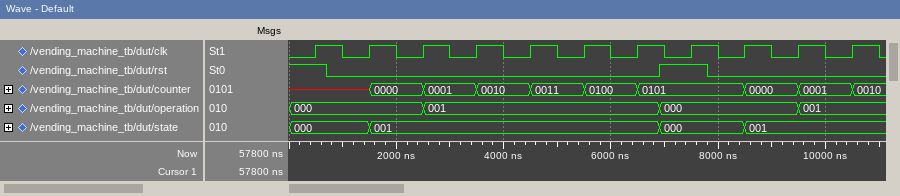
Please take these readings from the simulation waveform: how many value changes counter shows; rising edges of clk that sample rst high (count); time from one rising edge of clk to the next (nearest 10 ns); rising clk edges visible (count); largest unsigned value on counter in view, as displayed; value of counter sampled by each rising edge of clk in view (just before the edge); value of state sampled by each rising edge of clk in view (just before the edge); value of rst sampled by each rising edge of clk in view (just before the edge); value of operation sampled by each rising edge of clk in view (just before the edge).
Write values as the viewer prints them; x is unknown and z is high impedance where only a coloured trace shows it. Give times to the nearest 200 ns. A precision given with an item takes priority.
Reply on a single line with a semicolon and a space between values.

9; 2; 1000 ns; 11; 0101; x, x, 0000, 0001, 0010, 0011, 0100, 0101, 0101, 0000, 0001; 000, 000, 001, 001, 001, 001, 001, 000, 000, 001, 001; 1 0 0 0 0 0 0 1 0 0 0; 000, 000, 000, 001, 001, 001, 001, 000, 000, 000, 001
